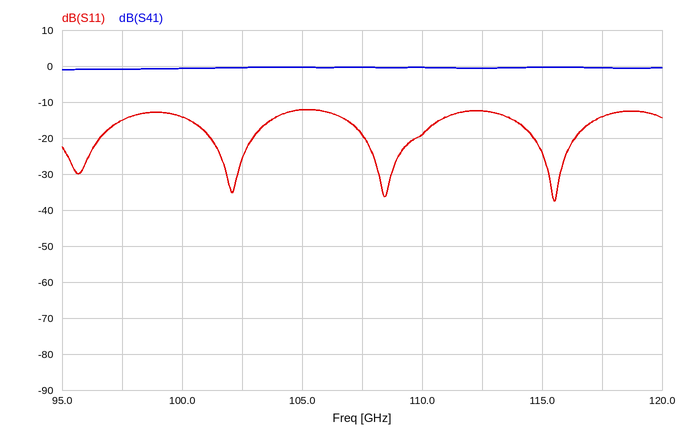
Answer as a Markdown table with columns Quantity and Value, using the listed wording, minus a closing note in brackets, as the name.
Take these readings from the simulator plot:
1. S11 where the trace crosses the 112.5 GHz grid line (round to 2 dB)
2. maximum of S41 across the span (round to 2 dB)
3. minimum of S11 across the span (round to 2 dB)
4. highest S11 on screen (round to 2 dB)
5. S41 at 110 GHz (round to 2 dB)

| Quantity | Value |
|---|---|
| S11 where the trace crosses the 112.5 GHz grid line | -12 dB |
| maximum of S41 across the span | 0 dB |
| minimum of S11 across the span | -38 dB |
| highest S11 on screen | -12 dB |
| S41 at 110 GHz | 0 dB |
